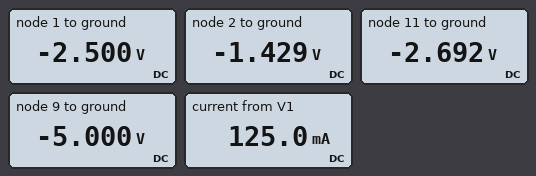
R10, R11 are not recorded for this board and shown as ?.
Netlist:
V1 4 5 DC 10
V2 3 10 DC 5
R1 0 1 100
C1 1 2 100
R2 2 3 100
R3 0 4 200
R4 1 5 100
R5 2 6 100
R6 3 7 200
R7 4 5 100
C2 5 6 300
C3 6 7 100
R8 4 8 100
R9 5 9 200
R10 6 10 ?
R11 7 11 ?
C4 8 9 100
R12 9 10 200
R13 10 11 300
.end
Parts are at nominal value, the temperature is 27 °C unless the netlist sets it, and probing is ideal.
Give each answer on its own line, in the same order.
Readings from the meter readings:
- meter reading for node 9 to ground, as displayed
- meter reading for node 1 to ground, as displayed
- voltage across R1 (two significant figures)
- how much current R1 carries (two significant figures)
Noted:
-5.000 V
-2.500 V
2.5 V
25 mA
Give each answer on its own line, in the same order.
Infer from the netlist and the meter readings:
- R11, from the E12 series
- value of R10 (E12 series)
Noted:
150 Ω
150 Ω
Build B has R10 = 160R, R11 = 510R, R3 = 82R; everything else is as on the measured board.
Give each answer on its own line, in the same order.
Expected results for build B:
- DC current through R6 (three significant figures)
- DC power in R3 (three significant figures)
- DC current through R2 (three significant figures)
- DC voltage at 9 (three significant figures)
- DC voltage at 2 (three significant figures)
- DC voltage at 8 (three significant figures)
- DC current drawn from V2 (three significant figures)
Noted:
4.95 mA
103 mW
13.9 mA
-7.09 V
-3.48 V
2.91 V
18.8 mA
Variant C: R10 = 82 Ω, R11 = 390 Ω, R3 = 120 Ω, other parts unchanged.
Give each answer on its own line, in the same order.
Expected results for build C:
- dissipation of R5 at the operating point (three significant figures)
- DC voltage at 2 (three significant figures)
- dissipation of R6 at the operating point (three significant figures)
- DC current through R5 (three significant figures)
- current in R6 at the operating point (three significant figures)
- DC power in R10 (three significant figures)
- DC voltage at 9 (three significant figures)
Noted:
31.4 mW
-3.02 V
6.31 mW
17.7 mA
5.62 mA
25.8 mW
-6.25 V
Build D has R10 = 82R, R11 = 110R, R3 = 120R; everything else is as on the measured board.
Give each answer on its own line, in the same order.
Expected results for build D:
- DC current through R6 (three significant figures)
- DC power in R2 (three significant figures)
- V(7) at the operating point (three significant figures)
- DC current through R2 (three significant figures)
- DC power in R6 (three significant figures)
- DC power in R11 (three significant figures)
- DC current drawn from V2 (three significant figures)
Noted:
8.20 mA
31.4 mW
-2.89 V
17.7 mA
13.4 mW
7.39 mW
25.9 mA
